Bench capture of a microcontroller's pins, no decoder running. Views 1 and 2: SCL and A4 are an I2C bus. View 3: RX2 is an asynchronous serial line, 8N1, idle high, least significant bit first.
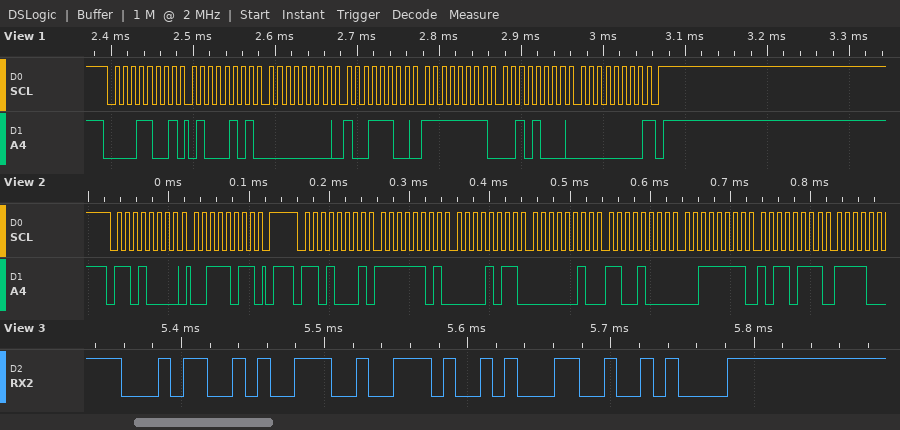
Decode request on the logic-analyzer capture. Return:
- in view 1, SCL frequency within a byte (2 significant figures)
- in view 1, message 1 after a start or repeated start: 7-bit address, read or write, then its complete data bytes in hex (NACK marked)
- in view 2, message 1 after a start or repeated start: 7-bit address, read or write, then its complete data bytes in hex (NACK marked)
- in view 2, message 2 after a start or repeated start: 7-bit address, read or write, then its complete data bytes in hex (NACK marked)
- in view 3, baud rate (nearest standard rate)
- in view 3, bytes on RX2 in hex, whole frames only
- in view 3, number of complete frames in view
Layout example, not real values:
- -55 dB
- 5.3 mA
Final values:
- 100 kHz
- 0x0C read: 45 00 9C FF 28 00 NACK
- 0x68 write: 3B
- 0x68 read: FD 0B 02 C8 3F B7
- 115200 baud
- 34 39 2E 31 0A
- 5
